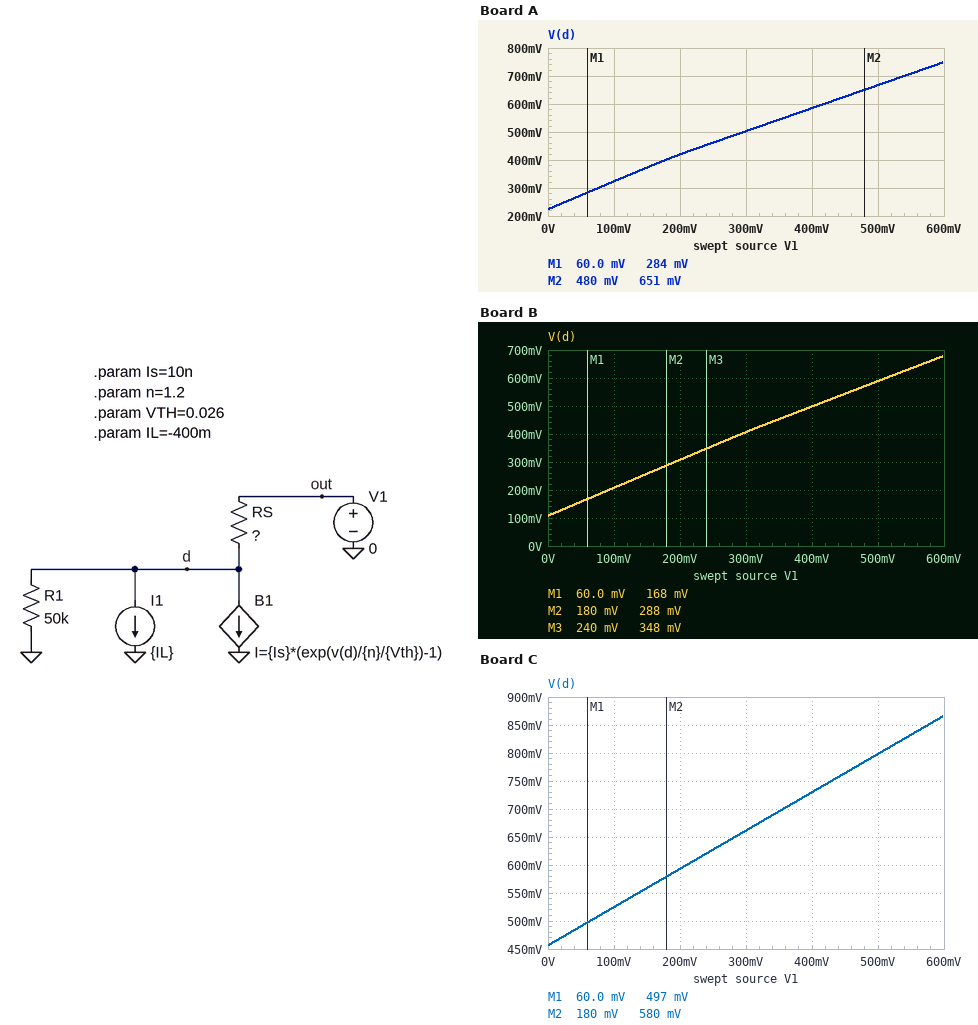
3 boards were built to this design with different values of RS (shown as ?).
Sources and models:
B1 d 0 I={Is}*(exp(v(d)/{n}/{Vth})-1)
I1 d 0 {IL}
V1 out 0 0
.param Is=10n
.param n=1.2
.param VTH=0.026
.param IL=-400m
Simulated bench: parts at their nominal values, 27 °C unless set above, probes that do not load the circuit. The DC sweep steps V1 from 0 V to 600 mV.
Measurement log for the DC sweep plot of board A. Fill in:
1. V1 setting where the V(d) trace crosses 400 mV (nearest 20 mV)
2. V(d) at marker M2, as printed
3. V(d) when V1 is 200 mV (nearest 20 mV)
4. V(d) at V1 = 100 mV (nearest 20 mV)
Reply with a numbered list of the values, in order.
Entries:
1. 180 mV
2. 651 mV
3. 420 mV
4. 320 mV
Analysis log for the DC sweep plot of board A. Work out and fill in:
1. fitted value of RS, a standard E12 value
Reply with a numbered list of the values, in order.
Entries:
1. 0.56 Ω
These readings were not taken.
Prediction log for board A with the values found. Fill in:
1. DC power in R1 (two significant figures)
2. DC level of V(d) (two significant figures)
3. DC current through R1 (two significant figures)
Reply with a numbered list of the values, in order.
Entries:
1. 1.0 µW
2. 220 mV
3. 4.5 µA
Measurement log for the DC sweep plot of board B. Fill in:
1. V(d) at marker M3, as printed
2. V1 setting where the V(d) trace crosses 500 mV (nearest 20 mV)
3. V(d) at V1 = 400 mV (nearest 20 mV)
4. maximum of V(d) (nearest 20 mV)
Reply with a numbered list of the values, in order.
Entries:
1. 348 mV
2. 400 mV
3. 500 mV
4. 680 mV
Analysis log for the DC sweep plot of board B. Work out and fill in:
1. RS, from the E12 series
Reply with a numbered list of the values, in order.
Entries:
1. 0.27 Ω
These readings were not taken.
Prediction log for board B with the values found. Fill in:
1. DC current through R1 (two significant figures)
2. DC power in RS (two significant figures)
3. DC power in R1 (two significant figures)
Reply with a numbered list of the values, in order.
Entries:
1. 2.2 µA
2. 43 mW
3. 230 nW
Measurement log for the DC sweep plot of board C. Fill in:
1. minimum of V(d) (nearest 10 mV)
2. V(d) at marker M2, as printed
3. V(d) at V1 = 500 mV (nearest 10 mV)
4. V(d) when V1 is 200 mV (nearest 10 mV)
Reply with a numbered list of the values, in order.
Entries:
1. 460 mV
2. 580 mV
3. 800 mV
4. 590 mV
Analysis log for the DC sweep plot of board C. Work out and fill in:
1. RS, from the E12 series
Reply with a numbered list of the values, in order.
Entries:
1. 1.2 Ω
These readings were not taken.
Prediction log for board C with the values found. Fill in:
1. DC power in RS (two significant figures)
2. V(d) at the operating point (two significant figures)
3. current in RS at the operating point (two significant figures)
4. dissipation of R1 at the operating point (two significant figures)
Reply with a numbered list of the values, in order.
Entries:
1. 170 mW
2. 460 mV
3. 380 mA
4. 4.2 µW
